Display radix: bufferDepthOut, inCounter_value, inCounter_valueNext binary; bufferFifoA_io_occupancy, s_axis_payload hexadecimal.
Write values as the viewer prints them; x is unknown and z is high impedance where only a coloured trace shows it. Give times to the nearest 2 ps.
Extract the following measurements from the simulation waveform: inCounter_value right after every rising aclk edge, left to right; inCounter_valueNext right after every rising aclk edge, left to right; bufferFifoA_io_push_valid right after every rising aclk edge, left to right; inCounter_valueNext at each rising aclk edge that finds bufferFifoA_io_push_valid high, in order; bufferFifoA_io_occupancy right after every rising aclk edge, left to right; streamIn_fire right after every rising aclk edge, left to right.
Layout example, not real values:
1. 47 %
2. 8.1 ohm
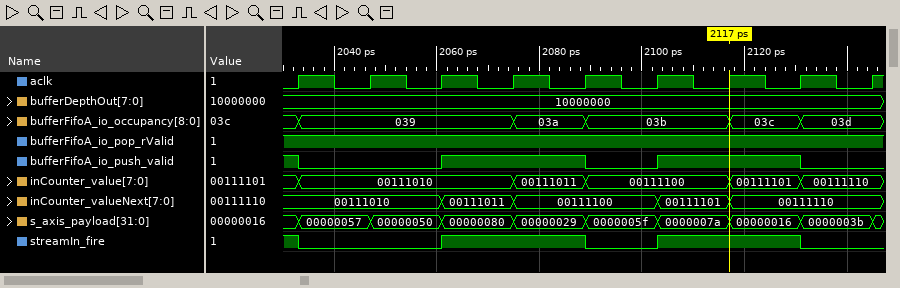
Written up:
1. 00111010, 00111010, 00111010, 00111011, 00111100, 00111100, 00111101, 00111110, 00111110
2. 00111010, 00111010, 00111011, 00111100, 00111100, 00111101, 00111110, 00111110, 00111110
3. 0 0 1 1 0 1 1 0 0
4. 00111010, 00111011, 00111100, 00111101, 00111110
5. 039, 039, 039, 03a, 03b, 03b, 03c, 03d, 03d
6. 0 0 1 1 0 1 1 0 0
